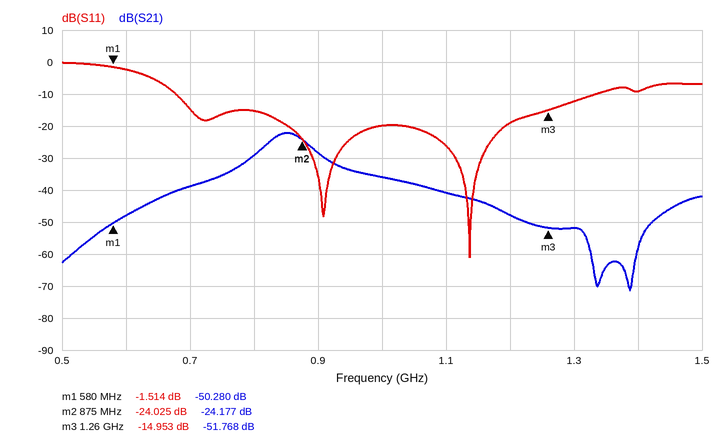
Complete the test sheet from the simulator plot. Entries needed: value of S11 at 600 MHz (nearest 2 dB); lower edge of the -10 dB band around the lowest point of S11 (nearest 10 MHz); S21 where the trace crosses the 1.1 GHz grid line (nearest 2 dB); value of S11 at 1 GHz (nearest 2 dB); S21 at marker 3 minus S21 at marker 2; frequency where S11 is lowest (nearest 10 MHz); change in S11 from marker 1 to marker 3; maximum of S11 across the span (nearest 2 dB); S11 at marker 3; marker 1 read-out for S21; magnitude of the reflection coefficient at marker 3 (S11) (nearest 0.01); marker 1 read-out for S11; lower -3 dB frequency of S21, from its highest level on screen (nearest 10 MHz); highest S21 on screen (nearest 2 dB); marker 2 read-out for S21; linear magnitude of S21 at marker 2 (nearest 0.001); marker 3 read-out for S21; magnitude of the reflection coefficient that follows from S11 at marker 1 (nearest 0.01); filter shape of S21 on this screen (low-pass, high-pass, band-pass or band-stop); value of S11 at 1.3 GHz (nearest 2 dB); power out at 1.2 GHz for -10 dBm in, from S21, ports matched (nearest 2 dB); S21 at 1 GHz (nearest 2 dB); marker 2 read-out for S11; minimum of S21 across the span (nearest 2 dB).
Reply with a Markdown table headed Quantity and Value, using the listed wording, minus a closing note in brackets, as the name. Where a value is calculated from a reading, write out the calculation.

| Quantity | Value |
|---|---|
| value of S11 at 600 MHz | -2 dB |
| lower edge of the -10 dB band around the lowest point of S11 | 680 MHz |
| S21 where the trace crosses the 1.1 GHz grid line | -40 dB |
| value of S11 at 1 GHz | -20 dB |
| S21 at marker 3 minus S21 at marker 2 | -51.768 − (-24.177) = -27.591 dB |
| frequency where S11 is lowest | 1.14 GHz |
| change in S11 from marker 1 to marker 3 | -14.953 − (-1.514) = -13.439 dB |
| maximum of S11 across the span | 0 dB |
| S11 at marker 3 | -14.953 dB |
| marker 1 read-out for S21 | -50.280 dB |
| magnitude of the reflection coefficient at marker 3 (S11) | 10^(-14.953/20) ≈ 0.18 |
| marker 1 read-out for S11 | -1.514 dB |
| lower -3 dB frequency of S21, from its highest level on screen | 820 MHz |
| highest S21 on screen | -22 dB |
| marker 2 read-out for S21 | -24.177 dB |
| linear magnitude of S21 at marker 2 | 10^(-24.177/20) ≈ 0.062 |
| marker 3 read-out for S21 | -51.768 dB |
| magnitude of the reflection coefficient that follows from S11 at marker 1 | 10^(-1.514/20) ≈ 0.84 |
| filter shape of S21 on this screen | band-pass |
| value of S11 at 1.3 GHz | -12 dB |
| power out at 1.2 GHz for -10 dBm in, from S21, ports matched | -10 dBm + (-48 dB) = -58 dBm |
| S21 at 1 GHz | -36 dB |
| marker 2 read-out for S11 | -24.025 dB |
| minimum of S21 across the span | -72 dB |
